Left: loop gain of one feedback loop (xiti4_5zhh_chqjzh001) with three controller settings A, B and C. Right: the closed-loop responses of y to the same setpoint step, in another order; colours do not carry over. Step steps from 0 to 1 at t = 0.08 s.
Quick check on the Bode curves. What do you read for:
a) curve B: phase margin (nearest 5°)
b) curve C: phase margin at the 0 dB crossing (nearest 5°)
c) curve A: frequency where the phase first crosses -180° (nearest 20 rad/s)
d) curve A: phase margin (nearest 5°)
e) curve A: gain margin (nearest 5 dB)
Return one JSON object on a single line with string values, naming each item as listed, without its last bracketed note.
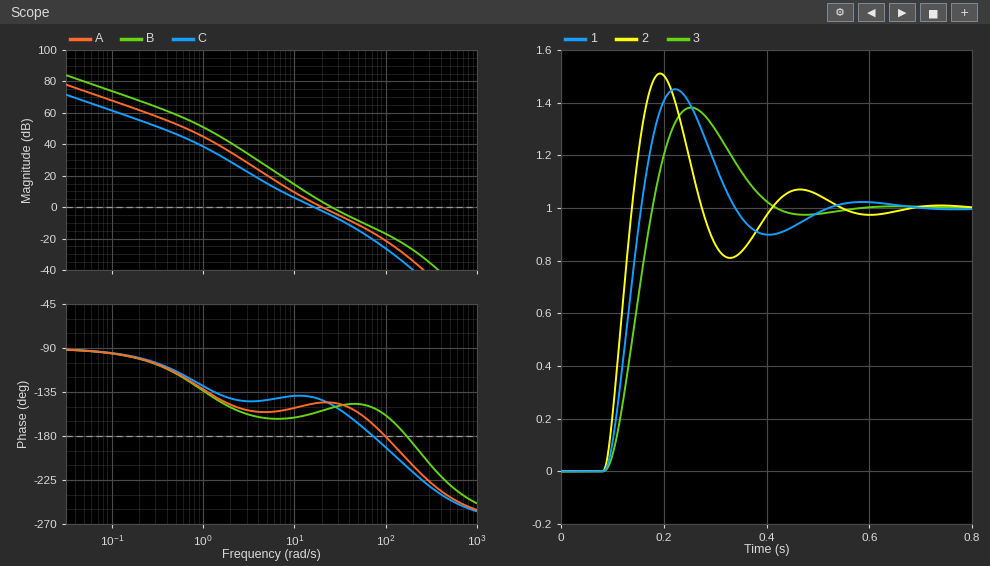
{"curve B: phase margin": "30°", "curve C: phase margin at the 0 dB crossing": "40°", "curve A: frequency where the phase first crosses -180°": "100 rad/s", "curve A: phase margin": "35°", "curve A: gain margin": "20 dB"}
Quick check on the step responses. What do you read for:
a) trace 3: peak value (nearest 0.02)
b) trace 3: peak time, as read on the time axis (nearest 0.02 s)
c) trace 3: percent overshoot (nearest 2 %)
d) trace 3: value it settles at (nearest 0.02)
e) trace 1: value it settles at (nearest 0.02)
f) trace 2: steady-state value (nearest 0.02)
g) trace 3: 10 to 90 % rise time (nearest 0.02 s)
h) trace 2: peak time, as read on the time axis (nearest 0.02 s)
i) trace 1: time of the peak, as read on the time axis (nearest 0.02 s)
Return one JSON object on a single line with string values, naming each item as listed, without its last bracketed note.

{"trace 3: peak value": "1.38", "trace 3: peak time, as read on the time axis": "0.26 s", "trace 3: percent overshoot": "38 %", "trace 3: value it settles at": "1.00", "trace 1: value it settles at": "1.00", "trace 2: steady-state value": "1.00", "trace 3: 10 to 90 % rise time": "0.06 s", "trace 2: peak time, as read on the time axis": "0.20 s", "trace 1: time of the peak, as read on the time axis": "0.22 s"}
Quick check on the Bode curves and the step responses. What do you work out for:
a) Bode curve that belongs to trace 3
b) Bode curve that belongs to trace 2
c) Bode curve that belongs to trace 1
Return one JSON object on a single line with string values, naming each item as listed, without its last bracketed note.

{"Bode curve that belongs to trace 3": "C", "Bode curve that belongs to trace 2": "B", "Bode curve that belongs to trace 1": "A"}
